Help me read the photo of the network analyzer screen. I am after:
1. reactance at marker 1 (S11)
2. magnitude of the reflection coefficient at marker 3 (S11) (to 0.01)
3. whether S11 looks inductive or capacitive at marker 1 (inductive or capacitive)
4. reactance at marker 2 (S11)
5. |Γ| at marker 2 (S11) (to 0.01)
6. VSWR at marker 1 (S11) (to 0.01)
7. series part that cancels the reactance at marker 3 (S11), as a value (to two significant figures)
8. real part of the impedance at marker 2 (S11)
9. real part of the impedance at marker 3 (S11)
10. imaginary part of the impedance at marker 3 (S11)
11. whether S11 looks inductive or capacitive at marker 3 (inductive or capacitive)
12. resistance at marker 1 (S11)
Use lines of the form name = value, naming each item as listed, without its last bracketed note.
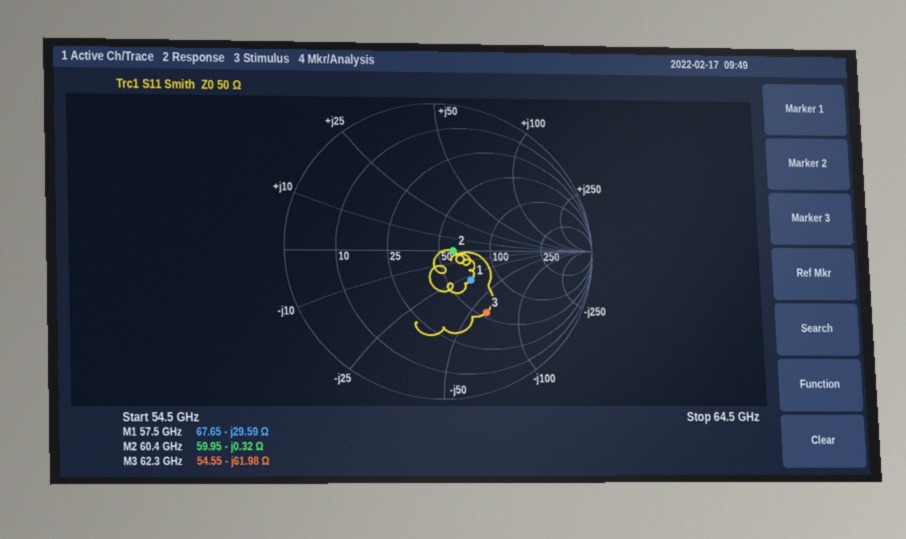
reactance at marker 1 = -29.59 Ω
magnitude of the reflection coefficient at marker 3 (S11) = 0.51
whether S11 looks inductive or capacitive at marker 1 = capacitive
reactance at marker 2 = -0.32 Ω
|Γ| at marker 2 (S11) = 0.09
VSWR at marker 1 (S11) = 1.79
series part that cancels the reactance at marker 3 (S11), as a value = 160 pH
real part of the impedance at marker 2 = 59.95 Ω
real part of the impedance at marker 3 = 54.55 Ω
imaginary part of the impedance at marker 3 = -61.98 Ω
whether S11 looks inductive or capacitive at marker 3 = capacitive
resistance at marker 1 = 67.65 Ω
